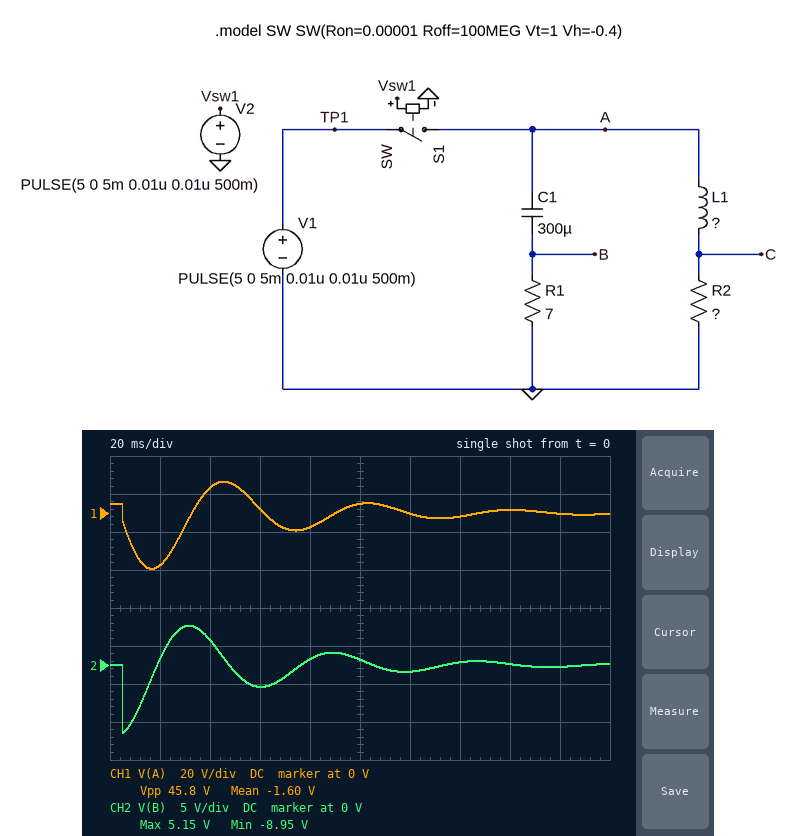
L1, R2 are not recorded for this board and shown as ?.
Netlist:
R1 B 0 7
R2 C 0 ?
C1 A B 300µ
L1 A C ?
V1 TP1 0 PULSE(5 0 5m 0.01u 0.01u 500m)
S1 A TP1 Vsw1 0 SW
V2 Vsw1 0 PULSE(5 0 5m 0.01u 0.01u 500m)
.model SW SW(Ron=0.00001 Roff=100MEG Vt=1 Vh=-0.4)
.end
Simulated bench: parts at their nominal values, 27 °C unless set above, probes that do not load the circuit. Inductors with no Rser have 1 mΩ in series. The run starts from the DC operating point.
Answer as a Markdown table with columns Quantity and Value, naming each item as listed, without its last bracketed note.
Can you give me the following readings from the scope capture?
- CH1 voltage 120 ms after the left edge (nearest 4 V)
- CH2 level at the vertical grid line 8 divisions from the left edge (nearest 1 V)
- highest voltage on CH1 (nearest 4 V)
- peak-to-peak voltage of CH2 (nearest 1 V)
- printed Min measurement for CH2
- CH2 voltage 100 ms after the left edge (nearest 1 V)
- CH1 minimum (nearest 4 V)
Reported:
| Quantity | Value |
|---|---|
| CH1 voltage 120 ms after the left edge | 0 V |
| CH2 level at the vertical grid line 8 divisions from the left edge | 0 V |
| highest voltage on CH1 | 16 V |
| peak-to-peak voltage of CH2 | 14 V |
| printed Min measurement for CH2 | -8.95 V |
| CH2 voltage 100 ms after the left edge | 1 V |
| CH1 minimum | -28 V |
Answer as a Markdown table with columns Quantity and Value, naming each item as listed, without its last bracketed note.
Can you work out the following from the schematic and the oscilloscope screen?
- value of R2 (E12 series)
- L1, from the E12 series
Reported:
| Quantity | Value |
|---|---|
| value of R2 | 3.9 Ω |
| L1, from the E12 series | 270 mH |
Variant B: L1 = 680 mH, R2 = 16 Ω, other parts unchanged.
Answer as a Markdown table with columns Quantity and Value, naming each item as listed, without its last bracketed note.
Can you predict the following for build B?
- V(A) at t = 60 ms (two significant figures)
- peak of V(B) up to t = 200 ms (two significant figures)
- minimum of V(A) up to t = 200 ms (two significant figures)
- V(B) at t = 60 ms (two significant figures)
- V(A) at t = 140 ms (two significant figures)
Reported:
| Quantity | Value |
|---|---|
| V(A) at t = 60 ms | 2.2 V |
| peak of V(B) up to t = 200 ms | 1.0 V |
| minimum of V(A) up to t = 200 ms | -9.7 V |
| V(B) at t = 60 ms | 760 mV |
| V(A) at t = 140 ms | -640 mV |
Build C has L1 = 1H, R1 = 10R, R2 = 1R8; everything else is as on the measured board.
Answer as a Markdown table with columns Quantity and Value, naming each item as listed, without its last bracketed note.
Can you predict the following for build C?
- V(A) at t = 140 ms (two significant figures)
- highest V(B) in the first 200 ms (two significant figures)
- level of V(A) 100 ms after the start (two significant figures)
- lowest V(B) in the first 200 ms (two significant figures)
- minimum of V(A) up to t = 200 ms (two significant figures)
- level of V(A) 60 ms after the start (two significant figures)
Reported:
| Quantity | Value |
|---|---|
| V(A) at t = 140 ms | -72 V |
| highest V(B) in the first 200 ms | 20 V |
| level of V(A) 100 ms after the start | 58 V |
| lowest V(B) in the first 200 ms | -28 V |
| minimum of V(A) up to t = 200 ms | -140 V |
| level of V(A) 60 ms after the start | 18 V |
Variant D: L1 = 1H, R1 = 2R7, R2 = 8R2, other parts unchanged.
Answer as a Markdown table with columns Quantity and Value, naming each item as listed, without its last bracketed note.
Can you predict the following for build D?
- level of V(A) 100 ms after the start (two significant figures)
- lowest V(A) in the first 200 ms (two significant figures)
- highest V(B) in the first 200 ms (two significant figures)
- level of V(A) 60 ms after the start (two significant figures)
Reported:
| Quantity | Value |
|---|---|
| level of V(A) 100 ms after the start | 17 V |
| lowest V(A) in the first 200 ms | -30 V |
| highest V(B) in the first 200 ms | 1.2 V |
| level of V(A) 60 ms after the start | -2.0 V |
